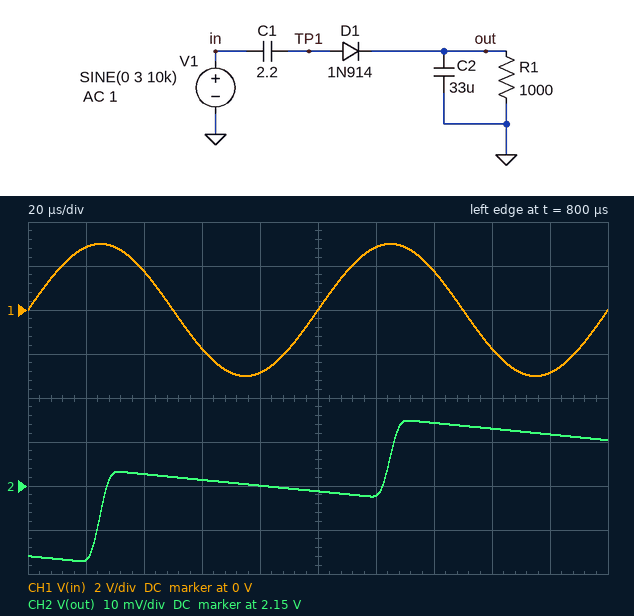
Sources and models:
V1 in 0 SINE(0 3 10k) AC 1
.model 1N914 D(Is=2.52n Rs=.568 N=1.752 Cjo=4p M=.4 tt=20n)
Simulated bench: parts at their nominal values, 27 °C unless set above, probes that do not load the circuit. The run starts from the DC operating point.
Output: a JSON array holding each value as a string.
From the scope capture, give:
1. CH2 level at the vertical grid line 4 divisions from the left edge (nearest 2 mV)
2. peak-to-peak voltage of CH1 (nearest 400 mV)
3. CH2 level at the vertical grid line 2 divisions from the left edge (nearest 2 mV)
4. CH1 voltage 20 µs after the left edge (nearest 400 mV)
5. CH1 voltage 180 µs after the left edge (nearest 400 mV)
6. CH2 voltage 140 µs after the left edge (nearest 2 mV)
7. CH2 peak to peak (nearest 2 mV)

["2.150 V", "6.0 V", "2.152 V", "2.8 V", "-2.8 V", "2.164 V", "32 mV"]
